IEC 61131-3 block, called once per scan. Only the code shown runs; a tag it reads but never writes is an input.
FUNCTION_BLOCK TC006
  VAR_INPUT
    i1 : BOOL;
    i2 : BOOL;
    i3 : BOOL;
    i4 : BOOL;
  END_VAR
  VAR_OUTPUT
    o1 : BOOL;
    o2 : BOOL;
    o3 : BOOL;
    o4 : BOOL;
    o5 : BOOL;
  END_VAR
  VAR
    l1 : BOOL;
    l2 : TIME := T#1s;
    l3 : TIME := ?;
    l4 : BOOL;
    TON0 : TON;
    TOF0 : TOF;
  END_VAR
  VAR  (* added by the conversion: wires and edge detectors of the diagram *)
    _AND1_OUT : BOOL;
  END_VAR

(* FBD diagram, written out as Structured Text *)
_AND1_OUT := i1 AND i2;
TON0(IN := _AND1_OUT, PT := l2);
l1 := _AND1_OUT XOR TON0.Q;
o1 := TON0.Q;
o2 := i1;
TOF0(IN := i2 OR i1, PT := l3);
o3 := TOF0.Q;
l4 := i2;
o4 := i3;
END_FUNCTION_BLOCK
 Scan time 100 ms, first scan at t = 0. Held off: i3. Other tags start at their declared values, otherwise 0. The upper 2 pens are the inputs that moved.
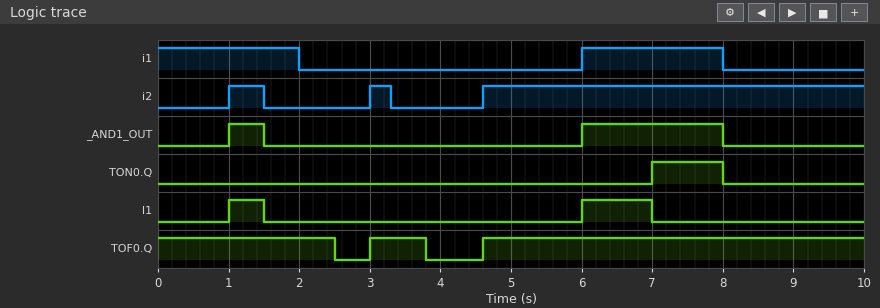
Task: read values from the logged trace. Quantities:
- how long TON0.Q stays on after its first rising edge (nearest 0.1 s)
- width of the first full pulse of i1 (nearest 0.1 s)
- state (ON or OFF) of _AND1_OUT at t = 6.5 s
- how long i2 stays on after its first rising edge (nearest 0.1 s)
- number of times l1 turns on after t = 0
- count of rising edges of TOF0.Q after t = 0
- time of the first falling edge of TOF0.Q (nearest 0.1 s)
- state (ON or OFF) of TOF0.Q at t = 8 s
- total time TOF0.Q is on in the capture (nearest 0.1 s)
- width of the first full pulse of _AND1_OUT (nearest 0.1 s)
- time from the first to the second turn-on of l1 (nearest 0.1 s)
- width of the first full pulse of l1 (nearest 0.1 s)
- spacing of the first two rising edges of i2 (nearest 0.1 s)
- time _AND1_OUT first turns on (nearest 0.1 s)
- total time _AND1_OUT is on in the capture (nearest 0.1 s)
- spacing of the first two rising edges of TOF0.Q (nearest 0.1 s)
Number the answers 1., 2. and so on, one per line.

1. 1.0 s
2. 2.0 s
3. ON
4. 0.5 s
5. 2
6. 2
7. 2.5 s
8. ON
9. 8.7 s
10. 0.5 s
11. 5.0 s
12. 0.5 s
13. 2.0 s
14. 1.0 s
15. 2.5 s
16. 1.6 s
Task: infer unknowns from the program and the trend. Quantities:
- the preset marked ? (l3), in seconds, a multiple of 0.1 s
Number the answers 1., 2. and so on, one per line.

1. 0.5 s
